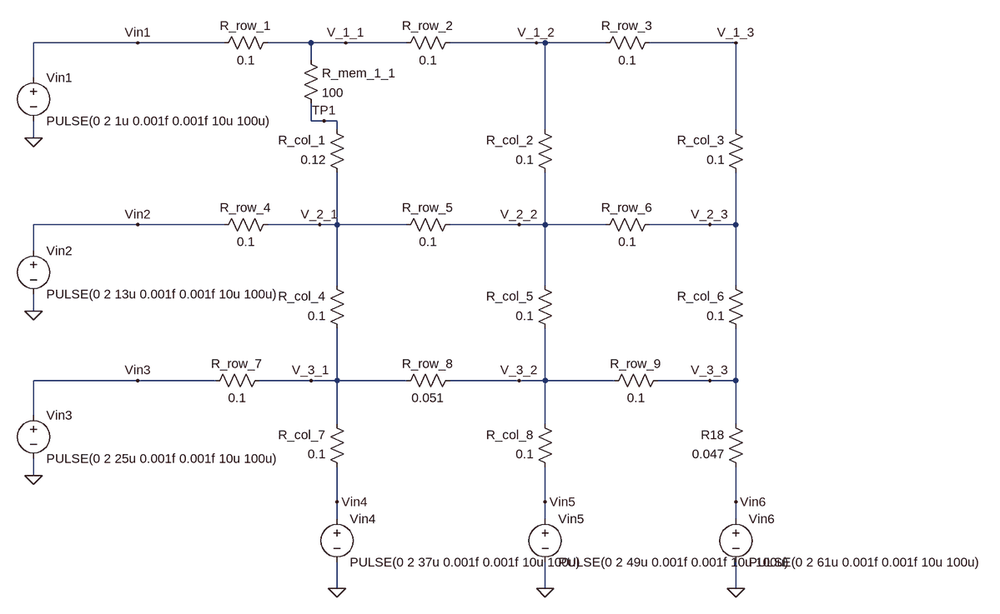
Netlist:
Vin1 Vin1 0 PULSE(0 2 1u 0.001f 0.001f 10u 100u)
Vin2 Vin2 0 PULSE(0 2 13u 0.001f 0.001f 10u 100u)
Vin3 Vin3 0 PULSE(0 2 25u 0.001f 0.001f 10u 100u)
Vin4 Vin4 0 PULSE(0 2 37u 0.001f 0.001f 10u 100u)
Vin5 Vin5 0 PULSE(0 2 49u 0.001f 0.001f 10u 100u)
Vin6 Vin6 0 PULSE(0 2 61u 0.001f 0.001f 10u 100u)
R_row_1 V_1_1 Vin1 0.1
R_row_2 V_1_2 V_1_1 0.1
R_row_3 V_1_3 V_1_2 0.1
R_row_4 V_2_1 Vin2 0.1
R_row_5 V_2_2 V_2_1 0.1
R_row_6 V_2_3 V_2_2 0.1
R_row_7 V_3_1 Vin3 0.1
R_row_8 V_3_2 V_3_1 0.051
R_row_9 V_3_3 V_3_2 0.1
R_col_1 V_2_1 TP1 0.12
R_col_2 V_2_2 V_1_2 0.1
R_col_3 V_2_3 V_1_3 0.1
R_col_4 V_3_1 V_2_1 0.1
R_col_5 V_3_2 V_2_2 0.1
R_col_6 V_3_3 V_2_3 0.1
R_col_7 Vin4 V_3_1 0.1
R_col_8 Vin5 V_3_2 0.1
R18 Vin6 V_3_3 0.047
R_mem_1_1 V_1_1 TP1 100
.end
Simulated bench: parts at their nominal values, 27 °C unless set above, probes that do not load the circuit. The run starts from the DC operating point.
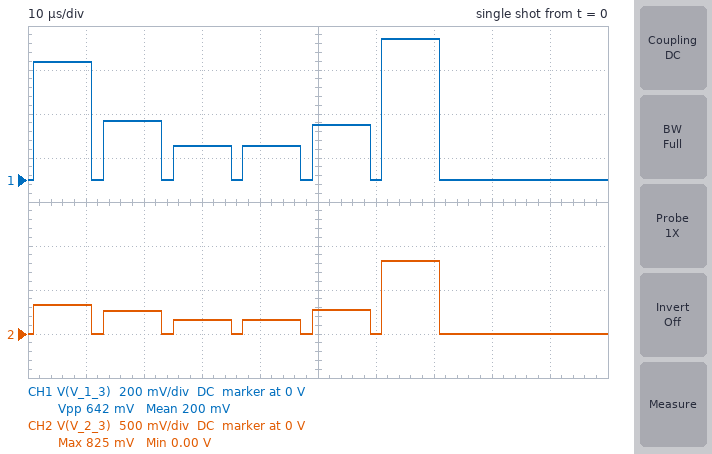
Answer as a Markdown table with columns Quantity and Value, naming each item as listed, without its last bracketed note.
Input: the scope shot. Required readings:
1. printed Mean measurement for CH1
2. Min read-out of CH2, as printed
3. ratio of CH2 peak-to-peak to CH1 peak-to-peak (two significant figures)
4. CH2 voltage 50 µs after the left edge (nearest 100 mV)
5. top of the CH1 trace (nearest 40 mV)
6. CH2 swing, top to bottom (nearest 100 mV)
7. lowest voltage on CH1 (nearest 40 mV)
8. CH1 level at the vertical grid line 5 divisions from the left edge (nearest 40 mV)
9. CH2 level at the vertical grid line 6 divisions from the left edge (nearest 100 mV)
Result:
| Quantity | Value |
|---|---|
| printed Mean measurement for CH1 | 200 mV |
| Min read-out of CH2, as printed | 0.00 V |
| ratio of CH2 peak-to-peak to CH1 peak-to-peak | 1.3 |
| CH2 voltage 50 µs after the left edge | 300 mV |
| top of the CH1 trace | 640 mV |
| CH2 swing, top to bottom | 800 mV |
| lowest voltage on CH1 | 0 V |
| CH1 level at the vertical grid line 5 divisions from the left edge | 240 mV |
| CH2 level at the vertical grid line 6 divisions from the left edge | 0 V |
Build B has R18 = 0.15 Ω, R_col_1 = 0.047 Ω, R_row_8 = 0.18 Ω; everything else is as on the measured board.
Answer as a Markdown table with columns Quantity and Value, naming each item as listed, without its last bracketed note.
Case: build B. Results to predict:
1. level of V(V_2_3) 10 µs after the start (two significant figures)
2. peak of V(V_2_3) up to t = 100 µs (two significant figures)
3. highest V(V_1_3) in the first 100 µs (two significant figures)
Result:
| Quantity | Value |
|---|---|
| level of V(V_2_3) 10 µs after the start | 390 mV |
| peak of V(V_2_3) up to t = 100 µs | 510 mV |
| highest V(V_1_3) in the first 100 µs | 590 mV |
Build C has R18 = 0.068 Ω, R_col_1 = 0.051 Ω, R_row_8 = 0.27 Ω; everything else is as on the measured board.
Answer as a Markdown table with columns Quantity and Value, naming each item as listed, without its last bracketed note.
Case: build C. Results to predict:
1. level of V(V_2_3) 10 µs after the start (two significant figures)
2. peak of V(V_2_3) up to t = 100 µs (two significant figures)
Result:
| Quantity | Value |
|---|---|
| level of V(V_2_3) 10 µs after the start | 350 mV |
| peak of V(V_2_3) up to t = 100 µs | 760 mV |
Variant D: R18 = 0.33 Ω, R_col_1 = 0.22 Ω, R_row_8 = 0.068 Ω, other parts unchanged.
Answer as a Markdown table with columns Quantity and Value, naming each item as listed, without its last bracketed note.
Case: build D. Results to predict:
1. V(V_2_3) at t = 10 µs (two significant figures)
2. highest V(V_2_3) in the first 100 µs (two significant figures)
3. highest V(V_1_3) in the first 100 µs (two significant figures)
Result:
| Quantity | Value |
|---|---|
| V(V_2_3) at t = 10 µs | 420 mV |
| highest V(V_2_3) in the first 100 µs | 470 mV |
| highest V(V_1_3) in the first 100 µs | 610 mV |
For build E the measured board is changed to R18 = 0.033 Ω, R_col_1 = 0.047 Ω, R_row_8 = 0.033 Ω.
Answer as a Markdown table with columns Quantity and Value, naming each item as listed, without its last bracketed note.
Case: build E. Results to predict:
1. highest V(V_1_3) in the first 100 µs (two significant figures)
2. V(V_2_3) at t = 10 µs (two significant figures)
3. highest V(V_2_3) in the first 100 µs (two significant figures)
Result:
| Quantity | Value |
|---|---|
| highest V(V_1_3) in the first 100 µs | 700 mV |
| V(V_2_3) at t = 10 µs | 310 mV |
| highest V(V_2_3) in the first 100 µs | 910 mV |
